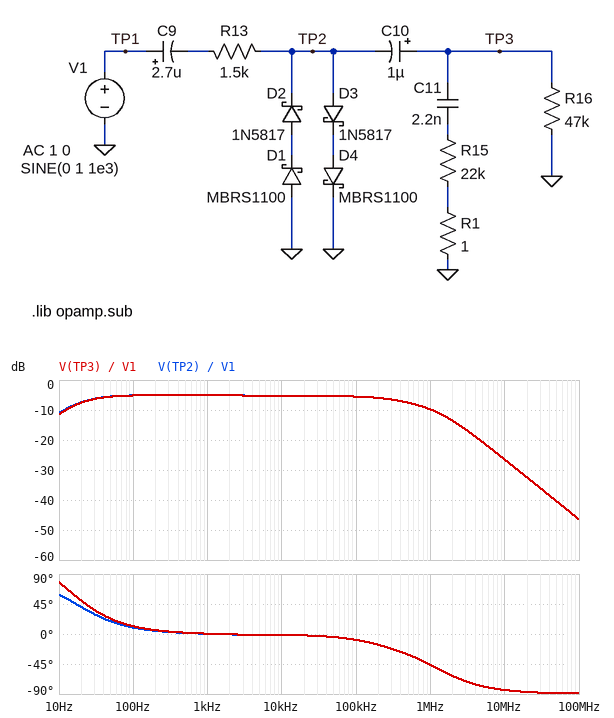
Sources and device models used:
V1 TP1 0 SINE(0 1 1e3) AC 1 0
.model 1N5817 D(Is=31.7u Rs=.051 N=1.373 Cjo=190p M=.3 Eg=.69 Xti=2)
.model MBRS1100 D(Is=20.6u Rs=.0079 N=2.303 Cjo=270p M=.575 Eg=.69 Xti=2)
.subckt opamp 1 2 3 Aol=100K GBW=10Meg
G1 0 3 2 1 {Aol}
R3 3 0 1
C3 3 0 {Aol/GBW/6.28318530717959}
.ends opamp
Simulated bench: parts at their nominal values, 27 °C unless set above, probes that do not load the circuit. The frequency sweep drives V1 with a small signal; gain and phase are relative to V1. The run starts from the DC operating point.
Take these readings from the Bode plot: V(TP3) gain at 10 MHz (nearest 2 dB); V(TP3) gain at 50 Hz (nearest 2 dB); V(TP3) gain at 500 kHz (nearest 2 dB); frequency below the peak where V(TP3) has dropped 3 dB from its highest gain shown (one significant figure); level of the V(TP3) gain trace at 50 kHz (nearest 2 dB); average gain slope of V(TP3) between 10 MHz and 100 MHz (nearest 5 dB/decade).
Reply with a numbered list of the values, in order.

1. -26 dB
2. -6 dB
3. -8 dB
4. 20 Hz
5. -6 dB
6. -20 dB/decade
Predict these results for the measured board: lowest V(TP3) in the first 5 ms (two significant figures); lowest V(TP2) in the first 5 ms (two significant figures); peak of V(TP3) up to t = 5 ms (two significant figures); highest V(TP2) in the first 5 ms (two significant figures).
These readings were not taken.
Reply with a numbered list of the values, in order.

1. -290 mV
2. -290 mV
3. 280 mV
4. 280 mV
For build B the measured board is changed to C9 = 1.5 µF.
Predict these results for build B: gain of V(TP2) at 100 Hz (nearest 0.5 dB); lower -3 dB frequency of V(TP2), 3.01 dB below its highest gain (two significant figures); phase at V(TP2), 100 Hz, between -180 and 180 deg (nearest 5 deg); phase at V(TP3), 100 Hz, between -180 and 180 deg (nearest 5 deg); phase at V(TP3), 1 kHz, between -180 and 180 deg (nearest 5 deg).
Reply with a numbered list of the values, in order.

1. -5.5 dB
2. 31 Hz
3. 15 deg
4. 20 deg
5. 0 deg
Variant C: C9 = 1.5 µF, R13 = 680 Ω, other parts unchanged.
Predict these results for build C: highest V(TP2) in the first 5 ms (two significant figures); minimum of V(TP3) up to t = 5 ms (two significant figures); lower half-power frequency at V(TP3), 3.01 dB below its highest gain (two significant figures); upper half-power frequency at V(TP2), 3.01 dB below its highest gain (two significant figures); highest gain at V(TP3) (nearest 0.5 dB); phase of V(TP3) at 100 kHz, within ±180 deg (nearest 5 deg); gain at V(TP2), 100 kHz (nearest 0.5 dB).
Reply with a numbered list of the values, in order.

1. 350 mV
2. -360 mV
3. 41 Hz
4. 1.2 MHz
5. -2.5 dB
6. -5 deg
7. -3.0 dB
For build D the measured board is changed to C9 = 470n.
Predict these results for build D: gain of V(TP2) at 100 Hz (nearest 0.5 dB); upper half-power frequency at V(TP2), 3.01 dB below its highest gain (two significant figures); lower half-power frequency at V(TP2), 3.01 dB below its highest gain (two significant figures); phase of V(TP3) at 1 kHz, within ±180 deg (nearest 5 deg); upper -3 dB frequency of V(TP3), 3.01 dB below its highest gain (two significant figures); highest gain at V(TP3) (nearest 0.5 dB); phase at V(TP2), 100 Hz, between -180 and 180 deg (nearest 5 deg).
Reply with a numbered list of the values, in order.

1. -8.0 dB
2. 610 kHz
3. 97 Hz
4. 5 deg
5. 620 kHz
6. -5.0 dB
7. 45 deg
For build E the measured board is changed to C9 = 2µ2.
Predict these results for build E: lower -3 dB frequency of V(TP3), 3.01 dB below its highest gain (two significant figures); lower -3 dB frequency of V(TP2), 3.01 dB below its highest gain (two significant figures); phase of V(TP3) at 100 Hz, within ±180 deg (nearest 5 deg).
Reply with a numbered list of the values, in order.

1. 22 Hz
2. 21 Hz
3. 15 deg
